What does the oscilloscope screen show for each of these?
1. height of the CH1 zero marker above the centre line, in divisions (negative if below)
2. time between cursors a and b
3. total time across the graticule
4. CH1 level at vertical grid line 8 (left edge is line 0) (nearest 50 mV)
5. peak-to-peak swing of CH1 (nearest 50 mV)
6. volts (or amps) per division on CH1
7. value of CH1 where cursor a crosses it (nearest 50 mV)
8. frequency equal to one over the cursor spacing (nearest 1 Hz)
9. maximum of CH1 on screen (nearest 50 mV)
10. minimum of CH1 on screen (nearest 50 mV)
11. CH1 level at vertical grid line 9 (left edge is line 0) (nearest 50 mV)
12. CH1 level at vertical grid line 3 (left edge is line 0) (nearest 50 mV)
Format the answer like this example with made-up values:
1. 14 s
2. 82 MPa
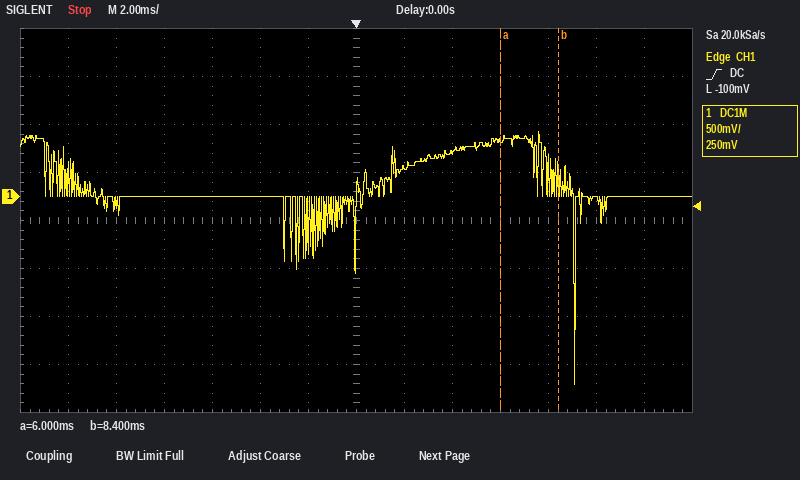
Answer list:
1. +0.5 div
2. 2.4 ms
3. 28 ms
4. 300 mV
5. 2.65 V
6. 500 mV
7. 600 mV
8. 417 Hz
9. 700 mV
10. -1.95 V
11. 450 mV
12. 0 mV
